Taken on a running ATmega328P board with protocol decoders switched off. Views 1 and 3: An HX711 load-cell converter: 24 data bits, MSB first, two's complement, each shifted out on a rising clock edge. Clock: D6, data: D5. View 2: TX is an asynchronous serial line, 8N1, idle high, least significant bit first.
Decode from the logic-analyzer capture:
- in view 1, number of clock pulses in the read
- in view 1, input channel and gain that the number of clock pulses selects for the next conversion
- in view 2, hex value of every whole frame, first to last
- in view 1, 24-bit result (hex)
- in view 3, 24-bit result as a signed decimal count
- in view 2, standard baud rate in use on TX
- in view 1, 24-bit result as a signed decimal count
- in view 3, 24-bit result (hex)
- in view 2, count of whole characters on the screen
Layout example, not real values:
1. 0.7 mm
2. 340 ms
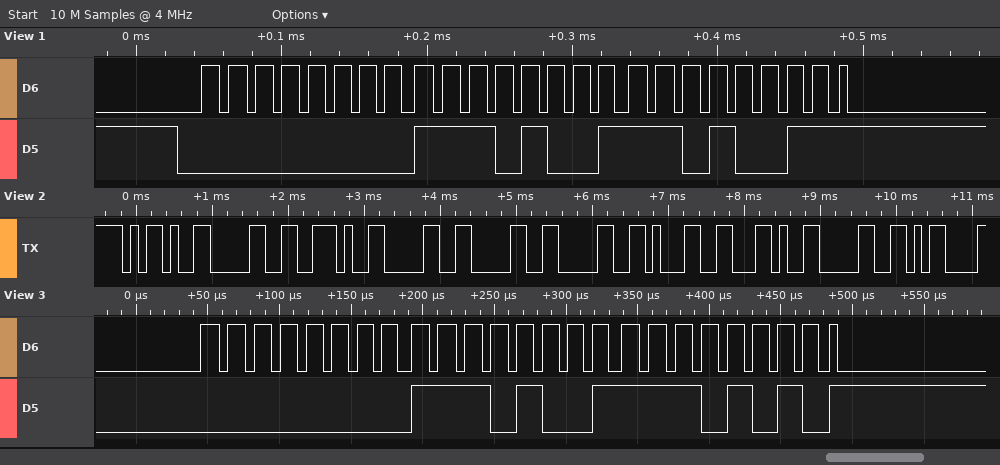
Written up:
1. 25
2. channel A, gain 128
3. 2D 30 2E 30 30 30 31 2C 30 0D
4. 0x00E9D3
5. 59882
6. 9600 baud
7. 59859
8. 0x00E9EA
9. 10
